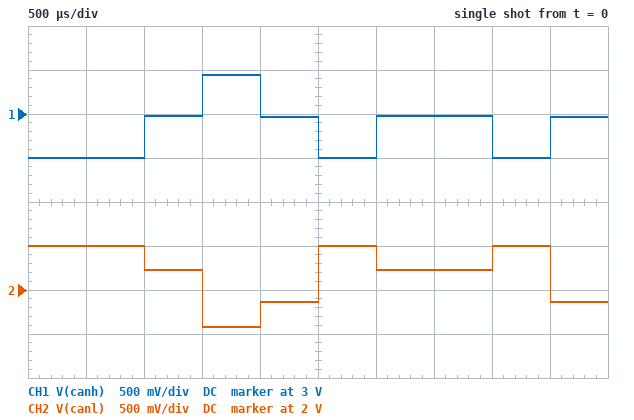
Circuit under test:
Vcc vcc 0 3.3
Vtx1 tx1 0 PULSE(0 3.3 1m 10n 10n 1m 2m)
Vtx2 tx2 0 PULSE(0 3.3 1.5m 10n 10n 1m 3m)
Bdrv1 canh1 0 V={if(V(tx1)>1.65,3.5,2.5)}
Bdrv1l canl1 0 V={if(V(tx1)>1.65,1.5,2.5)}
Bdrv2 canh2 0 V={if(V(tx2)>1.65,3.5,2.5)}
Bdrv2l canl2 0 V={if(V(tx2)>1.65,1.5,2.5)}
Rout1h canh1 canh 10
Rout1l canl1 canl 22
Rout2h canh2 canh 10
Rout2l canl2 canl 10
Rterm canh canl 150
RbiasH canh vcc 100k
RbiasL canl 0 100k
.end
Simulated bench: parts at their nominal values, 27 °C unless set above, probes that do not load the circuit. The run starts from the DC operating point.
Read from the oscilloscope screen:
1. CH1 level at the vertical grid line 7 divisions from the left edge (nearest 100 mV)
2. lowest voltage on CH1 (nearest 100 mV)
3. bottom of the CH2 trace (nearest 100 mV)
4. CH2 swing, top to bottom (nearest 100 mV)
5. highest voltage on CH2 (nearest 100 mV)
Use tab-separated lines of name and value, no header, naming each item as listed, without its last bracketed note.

CH1 level at the vertical grid line 7 divisions from the left edge	3.0 V
lowest voltage on CH1	2.5 V
bottom of the CH2 trace	1.6 V
CH2 swing, top to bottom	900 mV
highest voltage on CH2	2.5 V
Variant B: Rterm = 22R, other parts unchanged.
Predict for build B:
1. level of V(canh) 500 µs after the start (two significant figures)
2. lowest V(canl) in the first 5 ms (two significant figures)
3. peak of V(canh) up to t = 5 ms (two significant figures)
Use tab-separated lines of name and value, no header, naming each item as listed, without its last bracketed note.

level of V(canh) 500 µs after the start	2.5 V
lowest V(canl) in the first 5 ms	1.9 V
peak of V(canh) up to t = 5 ms	3.2 V
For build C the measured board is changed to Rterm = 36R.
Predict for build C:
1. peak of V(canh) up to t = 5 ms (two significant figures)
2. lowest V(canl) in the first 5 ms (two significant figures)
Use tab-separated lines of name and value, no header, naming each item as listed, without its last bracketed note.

peak of V(canh) up to t = 5 ms	3.3 V
lowest V(canl) in the first 5 ms	1.8 V
